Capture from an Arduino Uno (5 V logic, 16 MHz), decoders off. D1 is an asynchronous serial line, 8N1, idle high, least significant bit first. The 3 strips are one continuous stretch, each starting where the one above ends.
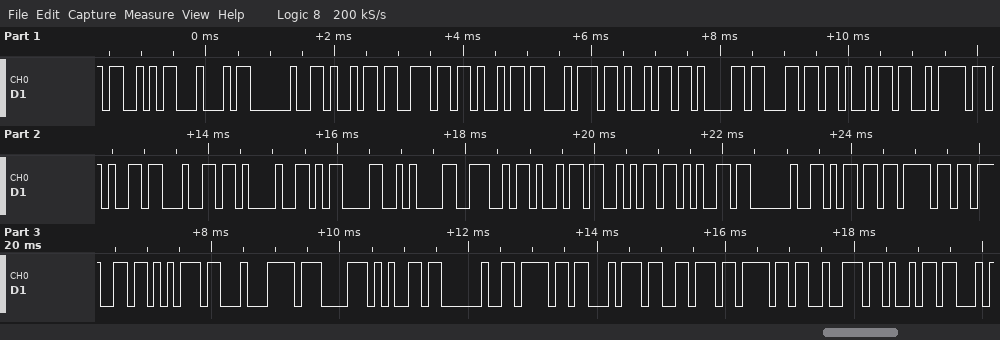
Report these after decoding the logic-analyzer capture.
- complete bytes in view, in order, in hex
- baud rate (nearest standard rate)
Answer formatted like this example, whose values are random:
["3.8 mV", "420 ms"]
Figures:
["53 44 20 69 6E 69 74 69 61 6C 69 7A 65 64 21 0D 0A 4E 69 6A 65 20 6D 6F 67 75 C4 87 65 20 6F 74 76 6F 72 69", "9600 baud"]
